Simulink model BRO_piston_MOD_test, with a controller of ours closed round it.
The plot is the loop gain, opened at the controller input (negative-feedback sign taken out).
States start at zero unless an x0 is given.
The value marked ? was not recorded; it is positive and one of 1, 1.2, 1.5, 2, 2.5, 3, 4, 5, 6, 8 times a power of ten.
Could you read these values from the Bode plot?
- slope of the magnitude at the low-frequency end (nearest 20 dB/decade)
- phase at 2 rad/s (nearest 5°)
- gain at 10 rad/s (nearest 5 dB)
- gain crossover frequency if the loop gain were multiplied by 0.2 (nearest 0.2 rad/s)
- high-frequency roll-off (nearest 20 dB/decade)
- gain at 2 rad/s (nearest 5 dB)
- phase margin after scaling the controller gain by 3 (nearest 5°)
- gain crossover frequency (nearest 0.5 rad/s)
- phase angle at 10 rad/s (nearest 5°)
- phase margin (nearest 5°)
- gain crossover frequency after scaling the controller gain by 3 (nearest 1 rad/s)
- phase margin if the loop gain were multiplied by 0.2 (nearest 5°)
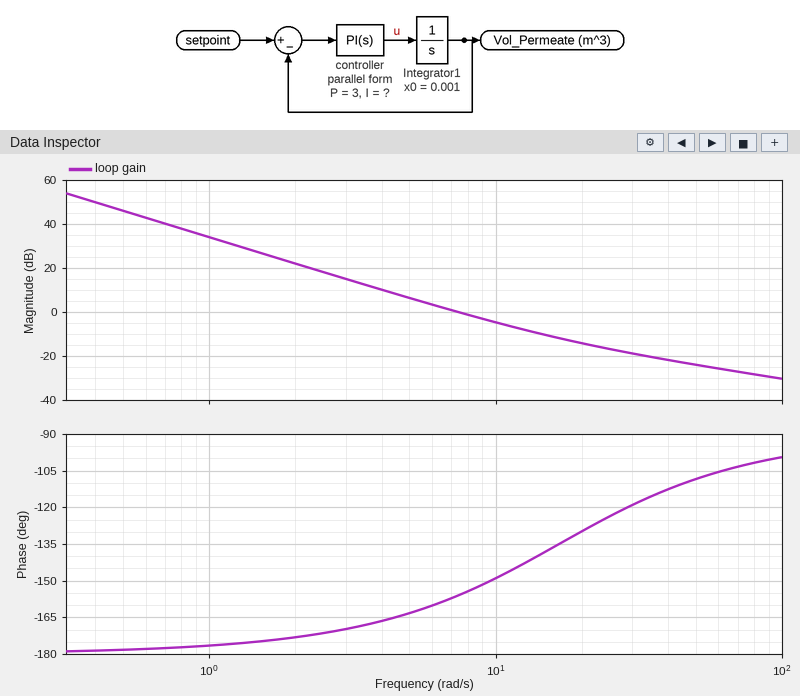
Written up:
-40 dB/decade
-175°
-5 dB
3.2 rad/s
-20 dB/decade
20 dB
40°
7.5 rad/s
-150°
25°
14 rad/s
10°
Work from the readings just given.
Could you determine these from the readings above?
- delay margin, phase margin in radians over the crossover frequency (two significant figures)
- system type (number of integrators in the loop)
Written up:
0.058 s
2
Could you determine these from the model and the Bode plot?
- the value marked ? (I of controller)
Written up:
50
